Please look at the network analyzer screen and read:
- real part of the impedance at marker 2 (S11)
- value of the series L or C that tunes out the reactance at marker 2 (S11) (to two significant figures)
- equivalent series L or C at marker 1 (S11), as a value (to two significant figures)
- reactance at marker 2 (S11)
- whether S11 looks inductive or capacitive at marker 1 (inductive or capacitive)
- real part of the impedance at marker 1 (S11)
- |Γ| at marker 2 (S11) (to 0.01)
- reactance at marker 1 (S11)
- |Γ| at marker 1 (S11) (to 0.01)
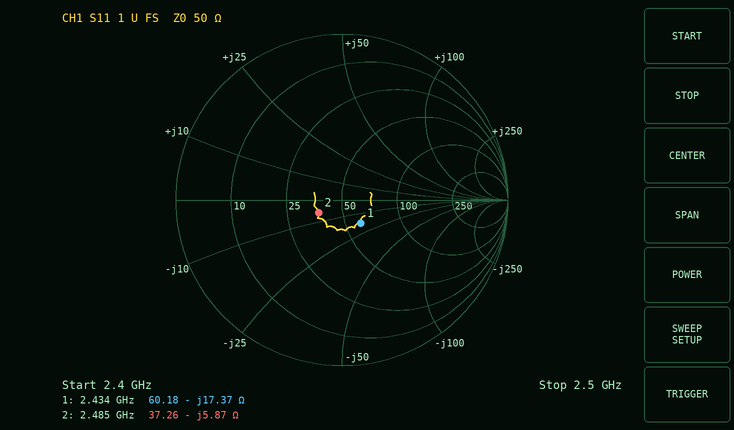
37.26 Ω
380 pH
3.8 pF
-5.87 Ω
capacitive
60.18 Ω
0.16
-17.37 Ω
0.18
